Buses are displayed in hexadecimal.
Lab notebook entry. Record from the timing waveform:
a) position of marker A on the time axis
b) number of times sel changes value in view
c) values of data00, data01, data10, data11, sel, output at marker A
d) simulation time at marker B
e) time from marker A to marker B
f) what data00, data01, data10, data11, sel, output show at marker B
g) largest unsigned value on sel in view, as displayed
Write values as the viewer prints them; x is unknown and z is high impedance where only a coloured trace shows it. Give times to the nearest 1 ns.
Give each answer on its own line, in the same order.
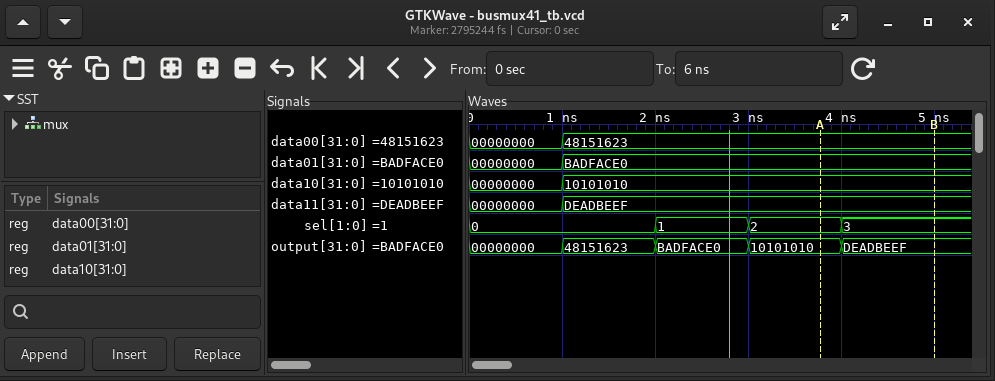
4 ns
3
data00=48151623, data01=BADFACE0, data10=10101010, data11=DEADBEEF, sel=2, output=10101010
5 ns
1 ns
data00=48151623, data01=BADFACE0, data10=10101010, data11=DEADBEEF, sel=3, output=DEADBEEF
3
